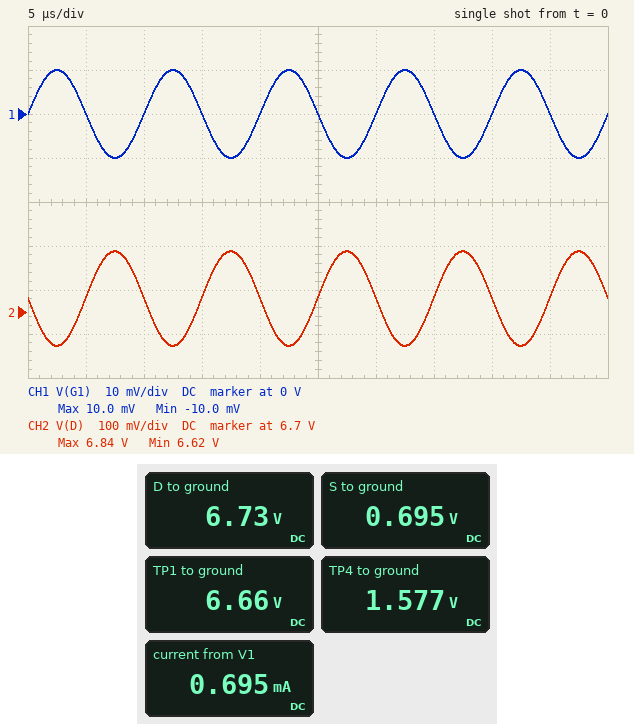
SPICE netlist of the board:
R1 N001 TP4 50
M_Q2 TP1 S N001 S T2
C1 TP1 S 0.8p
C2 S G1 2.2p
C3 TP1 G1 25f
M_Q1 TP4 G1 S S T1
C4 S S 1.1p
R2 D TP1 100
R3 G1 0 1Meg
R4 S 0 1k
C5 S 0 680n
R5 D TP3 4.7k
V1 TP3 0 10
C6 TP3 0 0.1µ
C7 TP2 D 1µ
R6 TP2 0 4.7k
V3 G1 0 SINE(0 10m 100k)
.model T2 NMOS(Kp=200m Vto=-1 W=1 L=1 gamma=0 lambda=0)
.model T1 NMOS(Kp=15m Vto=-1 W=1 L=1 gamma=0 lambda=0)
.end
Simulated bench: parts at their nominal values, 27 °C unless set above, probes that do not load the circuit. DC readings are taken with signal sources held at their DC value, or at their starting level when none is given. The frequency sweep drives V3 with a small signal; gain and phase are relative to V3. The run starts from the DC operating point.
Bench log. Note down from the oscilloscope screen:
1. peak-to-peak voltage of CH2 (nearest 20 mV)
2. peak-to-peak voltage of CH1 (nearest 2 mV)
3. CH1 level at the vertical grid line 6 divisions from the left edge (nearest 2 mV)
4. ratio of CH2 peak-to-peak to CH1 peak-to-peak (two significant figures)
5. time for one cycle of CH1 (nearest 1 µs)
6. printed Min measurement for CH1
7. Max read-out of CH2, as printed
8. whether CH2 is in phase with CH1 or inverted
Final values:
220 mV
20 mV
0 V
11
10 µs
-10.0 mV
6.84 V
inverted
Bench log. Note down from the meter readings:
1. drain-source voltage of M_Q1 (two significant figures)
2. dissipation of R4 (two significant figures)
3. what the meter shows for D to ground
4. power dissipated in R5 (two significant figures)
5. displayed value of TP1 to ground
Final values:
880 mV
480 µW
6.73 V
2.3 mW
6.66 V
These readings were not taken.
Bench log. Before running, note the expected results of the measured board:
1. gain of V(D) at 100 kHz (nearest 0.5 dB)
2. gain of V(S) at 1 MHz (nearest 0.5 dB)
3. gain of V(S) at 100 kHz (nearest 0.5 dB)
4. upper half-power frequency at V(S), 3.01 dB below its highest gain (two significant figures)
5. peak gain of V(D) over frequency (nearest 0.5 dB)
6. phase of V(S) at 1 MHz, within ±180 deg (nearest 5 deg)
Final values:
20.5 dB
-59.5 dB
-39.5 dB
1.3 kHz
20.5 dB
-90 deg
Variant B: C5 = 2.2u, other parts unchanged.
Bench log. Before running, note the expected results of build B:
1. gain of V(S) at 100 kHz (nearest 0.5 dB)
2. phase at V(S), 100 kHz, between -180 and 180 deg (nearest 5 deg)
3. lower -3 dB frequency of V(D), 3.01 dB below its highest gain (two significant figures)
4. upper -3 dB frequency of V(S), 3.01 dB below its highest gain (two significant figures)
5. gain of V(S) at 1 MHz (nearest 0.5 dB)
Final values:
-49.5 dB
-90 deg
390 Hz
400 Hz
-69.5 dB
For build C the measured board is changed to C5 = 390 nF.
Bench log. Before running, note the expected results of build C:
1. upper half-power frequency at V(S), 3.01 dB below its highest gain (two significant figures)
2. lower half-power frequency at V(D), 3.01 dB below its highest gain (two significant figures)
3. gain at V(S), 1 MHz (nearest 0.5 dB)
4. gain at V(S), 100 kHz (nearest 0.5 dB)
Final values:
2.3 kHz
2.2 kHz
-54.5 dB
-34.5 dB
